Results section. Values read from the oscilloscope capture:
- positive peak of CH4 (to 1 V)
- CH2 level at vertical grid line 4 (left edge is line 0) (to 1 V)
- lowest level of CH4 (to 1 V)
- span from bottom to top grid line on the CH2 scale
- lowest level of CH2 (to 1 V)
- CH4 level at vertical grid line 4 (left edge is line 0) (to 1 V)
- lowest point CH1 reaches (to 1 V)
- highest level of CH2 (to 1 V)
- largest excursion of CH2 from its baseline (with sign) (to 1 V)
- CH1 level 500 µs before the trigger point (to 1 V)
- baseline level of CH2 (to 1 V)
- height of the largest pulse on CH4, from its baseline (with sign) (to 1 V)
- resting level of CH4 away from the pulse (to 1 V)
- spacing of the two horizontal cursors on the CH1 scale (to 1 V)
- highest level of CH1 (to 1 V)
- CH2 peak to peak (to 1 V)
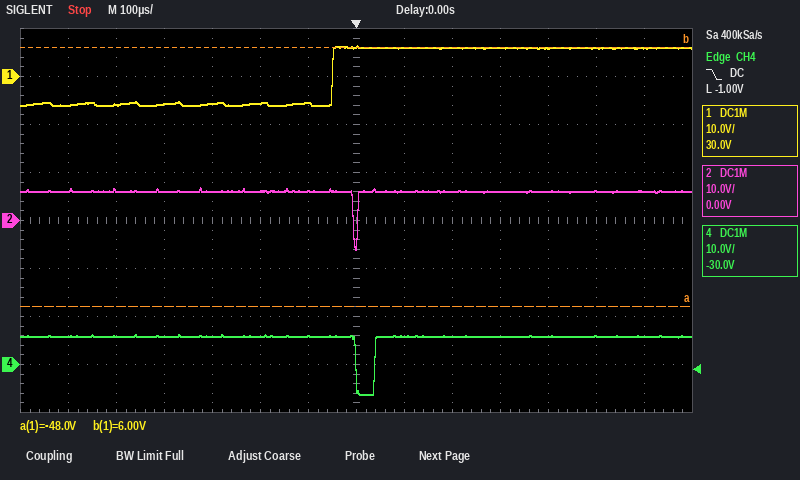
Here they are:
6 V
6 V
-6 V
80 V
-6 V
6 V
-6 V
7 V
-12 V
-6 V
6 V
-12 V
6 V
54 V
6 V
13 V
